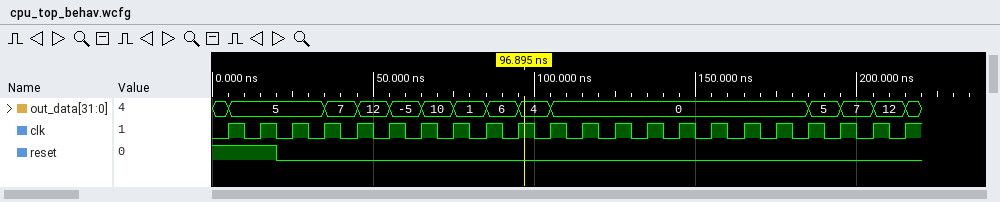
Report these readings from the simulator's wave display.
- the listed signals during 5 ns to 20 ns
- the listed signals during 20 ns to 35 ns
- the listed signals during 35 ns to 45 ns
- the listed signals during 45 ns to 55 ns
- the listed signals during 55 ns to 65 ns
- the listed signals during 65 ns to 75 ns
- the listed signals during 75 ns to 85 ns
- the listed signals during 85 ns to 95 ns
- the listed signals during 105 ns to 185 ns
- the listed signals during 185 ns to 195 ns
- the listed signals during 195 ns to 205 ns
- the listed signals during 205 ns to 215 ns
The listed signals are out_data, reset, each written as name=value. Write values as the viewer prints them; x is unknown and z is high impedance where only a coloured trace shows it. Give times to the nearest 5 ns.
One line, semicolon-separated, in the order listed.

out_data=5, reset=1; out_data=5, reset=0; out_data=7, reset=0; out_data=12, reset=0; out_data=-5, reset=0; out_data=10, reset=0; out_data=1, reset=0; out_data=6, reset=0; out_data=0, reset=0; out_data=5, reset=0; out_data=7, reset=0; out_data=12, reset=0
